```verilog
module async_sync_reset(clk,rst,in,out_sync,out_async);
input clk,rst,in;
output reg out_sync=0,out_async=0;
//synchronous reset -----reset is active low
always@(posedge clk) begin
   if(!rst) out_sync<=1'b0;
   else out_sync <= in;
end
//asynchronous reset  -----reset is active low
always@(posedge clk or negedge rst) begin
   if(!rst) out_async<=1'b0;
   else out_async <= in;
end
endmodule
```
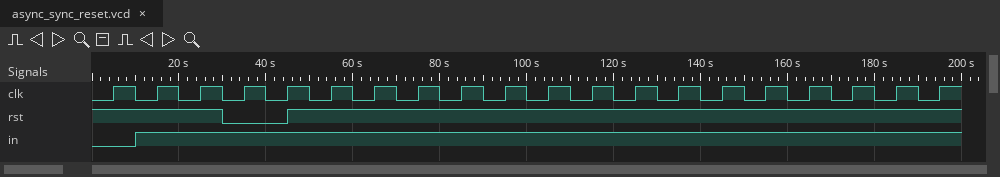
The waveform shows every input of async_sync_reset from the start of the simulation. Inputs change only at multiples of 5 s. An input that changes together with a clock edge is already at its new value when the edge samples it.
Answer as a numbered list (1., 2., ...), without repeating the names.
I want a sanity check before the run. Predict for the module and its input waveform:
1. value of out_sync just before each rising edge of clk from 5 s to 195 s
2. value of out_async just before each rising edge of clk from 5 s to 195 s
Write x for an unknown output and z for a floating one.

1. 0 0 1 1 0 1 1 1 1 1 1 1 1 1 1 1 1 1 1 1
2. 0 0 1 0 0 1 1 1 1 1 1 1 1 1 1 1 1 1 1 1
